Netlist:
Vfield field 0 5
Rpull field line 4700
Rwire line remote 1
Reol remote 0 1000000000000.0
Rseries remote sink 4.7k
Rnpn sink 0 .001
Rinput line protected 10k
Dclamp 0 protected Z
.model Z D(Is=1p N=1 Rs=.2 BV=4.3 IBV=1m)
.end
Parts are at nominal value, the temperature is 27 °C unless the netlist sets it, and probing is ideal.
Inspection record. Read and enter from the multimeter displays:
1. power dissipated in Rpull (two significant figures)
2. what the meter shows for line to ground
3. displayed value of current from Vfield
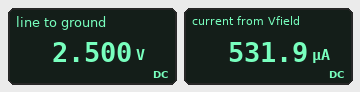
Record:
1.3 mW
2.500 V
531.9 µA
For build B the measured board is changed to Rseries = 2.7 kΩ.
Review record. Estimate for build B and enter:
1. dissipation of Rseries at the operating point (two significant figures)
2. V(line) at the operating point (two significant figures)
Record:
1.2 mW
1.8 V
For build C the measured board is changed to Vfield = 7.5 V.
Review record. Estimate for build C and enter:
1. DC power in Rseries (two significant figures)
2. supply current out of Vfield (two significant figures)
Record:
3.0 mW
800 µA
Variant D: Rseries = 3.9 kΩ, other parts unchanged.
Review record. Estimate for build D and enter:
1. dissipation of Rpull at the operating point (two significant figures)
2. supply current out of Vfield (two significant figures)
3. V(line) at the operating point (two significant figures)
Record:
1.6 mW
580 µA
2.3 V
